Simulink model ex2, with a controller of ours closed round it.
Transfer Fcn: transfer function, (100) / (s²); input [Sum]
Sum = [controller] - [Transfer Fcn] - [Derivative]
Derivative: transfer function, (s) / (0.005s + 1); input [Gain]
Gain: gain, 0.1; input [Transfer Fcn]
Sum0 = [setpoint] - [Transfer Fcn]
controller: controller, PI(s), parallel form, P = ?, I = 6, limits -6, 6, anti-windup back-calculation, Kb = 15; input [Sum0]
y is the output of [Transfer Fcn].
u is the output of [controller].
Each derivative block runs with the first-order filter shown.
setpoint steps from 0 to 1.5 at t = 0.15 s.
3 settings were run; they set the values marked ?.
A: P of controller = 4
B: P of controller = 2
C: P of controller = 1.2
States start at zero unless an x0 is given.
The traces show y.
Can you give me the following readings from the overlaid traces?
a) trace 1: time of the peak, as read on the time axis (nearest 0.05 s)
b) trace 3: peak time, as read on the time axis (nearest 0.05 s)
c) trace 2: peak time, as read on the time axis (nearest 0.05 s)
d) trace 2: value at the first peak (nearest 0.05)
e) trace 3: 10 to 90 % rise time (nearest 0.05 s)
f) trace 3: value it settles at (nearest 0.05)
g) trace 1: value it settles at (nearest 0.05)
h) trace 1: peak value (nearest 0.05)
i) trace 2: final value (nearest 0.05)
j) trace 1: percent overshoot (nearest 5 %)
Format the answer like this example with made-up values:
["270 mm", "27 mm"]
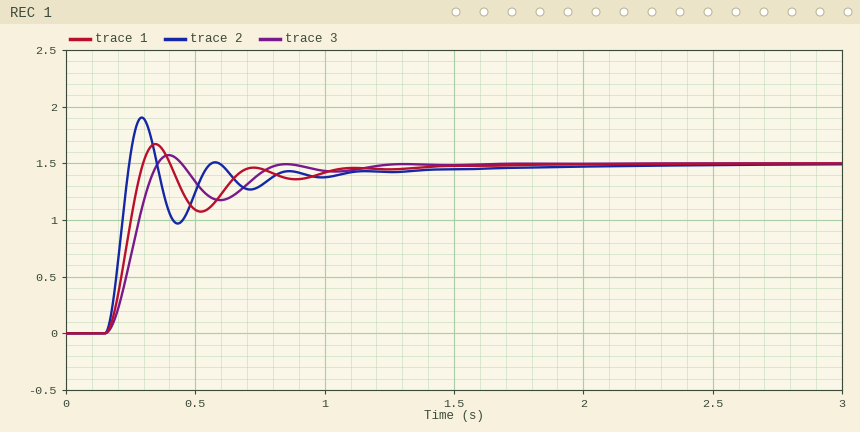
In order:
["0.35 s", "0.40 s", "0.30 s", "1.90", "0.15 s", "1.50", "1.50", "1.65", "1.50", "10 %"]
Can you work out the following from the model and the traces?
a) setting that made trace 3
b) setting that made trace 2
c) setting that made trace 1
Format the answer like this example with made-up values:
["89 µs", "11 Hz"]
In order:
["C", "A", "B"]
